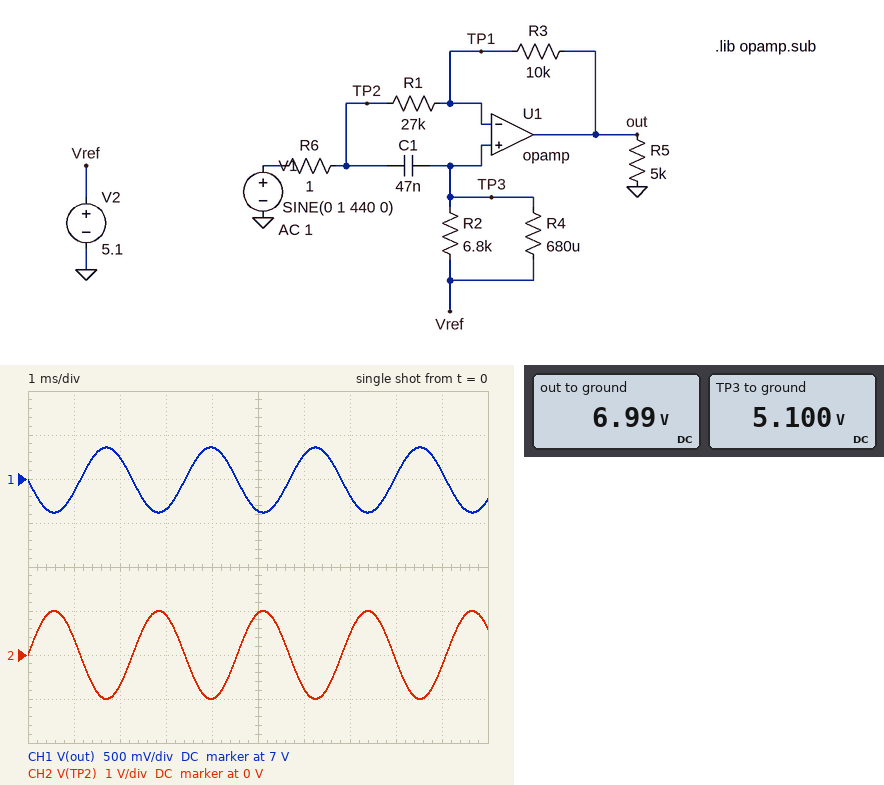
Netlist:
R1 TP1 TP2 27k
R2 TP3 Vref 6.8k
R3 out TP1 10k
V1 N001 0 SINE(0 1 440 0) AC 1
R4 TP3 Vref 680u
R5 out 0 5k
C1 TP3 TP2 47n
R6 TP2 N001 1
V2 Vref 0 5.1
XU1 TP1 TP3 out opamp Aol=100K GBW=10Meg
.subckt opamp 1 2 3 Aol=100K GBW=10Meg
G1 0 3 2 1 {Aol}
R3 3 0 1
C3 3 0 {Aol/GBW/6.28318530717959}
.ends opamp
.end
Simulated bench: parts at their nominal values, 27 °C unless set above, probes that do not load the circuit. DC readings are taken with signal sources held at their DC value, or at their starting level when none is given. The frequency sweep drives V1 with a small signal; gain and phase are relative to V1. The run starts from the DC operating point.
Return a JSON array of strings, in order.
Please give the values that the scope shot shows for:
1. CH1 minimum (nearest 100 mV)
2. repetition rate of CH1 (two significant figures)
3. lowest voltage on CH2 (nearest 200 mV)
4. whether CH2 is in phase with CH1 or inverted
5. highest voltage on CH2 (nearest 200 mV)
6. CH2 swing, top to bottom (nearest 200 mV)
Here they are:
["6.6 V", "440 Hz", "-1.0 V", "inverted", "1.0 V", "2.0 V"]
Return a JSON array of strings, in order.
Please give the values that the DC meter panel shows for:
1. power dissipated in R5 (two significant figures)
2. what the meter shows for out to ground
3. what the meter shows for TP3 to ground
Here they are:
["9.8 mW", "6.99 V", "5.100 V"]
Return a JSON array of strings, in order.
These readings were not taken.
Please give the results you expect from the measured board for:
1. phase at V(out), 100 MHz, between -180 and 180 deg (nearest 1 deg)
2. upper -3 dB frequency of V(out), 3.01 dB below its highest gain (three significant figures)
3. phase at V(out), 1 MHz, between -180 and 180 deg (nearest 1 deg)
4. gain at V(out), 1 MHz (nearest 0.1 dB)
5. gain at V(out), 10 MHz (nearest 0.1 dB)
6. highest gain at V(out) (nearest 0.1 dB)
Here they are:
["3 deg", "2.89 MHz", "156 deg", "-9.1 dB", "-23.1 dB", "-8.6 dB"]
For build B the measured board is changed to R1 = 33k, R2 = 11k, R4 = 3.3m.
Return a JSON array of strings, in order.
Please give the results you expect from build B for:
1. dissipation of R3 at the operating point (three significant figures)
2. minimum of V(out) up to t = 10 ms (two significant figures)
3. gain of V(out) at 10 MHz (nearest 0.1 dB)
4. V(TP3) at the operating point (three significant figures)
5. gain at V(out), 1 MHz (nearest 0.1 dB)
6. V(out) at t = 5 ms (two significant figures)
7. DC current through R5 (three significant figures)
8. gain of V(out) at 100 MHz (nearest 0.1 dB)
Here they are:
["239 µW", "6.3 V", "-24.6 dB", "5.10 V", "-10.8 dB", "6.4 V", "1.33 mA", "-61.7 dB"]
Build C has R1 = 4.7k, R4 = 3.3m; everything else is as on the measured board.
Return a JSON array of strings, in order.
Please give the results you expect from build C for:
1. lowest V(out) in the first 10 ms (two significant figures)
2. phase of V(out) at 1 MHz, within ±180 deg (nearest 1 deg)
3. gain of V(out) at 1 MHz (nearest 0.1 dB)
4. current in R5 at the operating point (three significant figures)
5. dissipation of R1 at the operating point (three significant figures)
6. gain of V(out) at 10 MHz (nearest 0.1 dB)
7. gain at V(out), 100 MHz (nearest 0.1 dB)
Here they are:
["14 V", "146 deg", "5.8 dB", "3.19 mA", "5.53 mW", "-13.7 dB", "-52.8 dB"]
